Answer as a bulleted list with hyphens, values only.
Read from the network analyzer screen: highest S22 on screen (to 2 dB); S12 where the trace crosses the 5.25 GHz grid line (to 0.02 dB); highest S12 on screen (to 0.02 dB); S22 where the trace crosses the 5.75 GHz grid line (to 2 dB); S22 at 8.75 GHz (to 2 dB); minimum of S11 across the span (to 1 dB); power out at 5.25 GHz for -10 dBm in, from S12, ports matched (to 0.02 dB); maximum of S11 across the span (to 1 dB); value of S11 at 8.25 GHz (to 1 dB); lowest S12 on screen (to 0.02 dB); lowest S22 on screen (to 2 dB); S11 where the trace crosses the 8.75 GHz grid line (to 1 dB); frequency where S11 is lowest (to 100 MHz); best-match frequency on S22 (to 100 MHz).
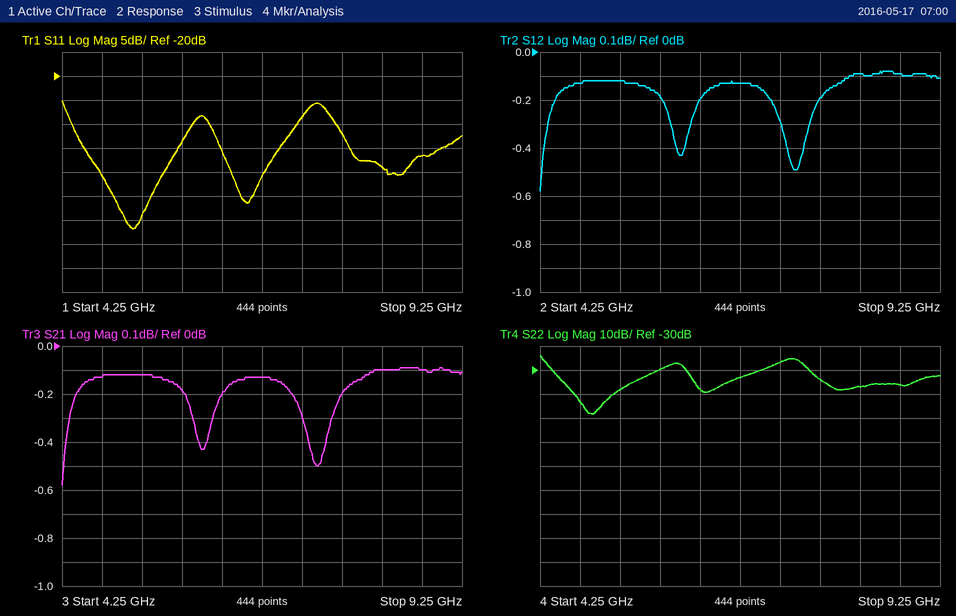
- -24 dB
- -0.12 dB
- -0.08 dB
- -30 dB
- -36 dB
- -52 dB
- -10.12 dBm
- -25 dB
- -39 dB
- -0.58 dB
- -48 dB
- -37 dB
- 5.1 GHz
- 4.9 GHz
